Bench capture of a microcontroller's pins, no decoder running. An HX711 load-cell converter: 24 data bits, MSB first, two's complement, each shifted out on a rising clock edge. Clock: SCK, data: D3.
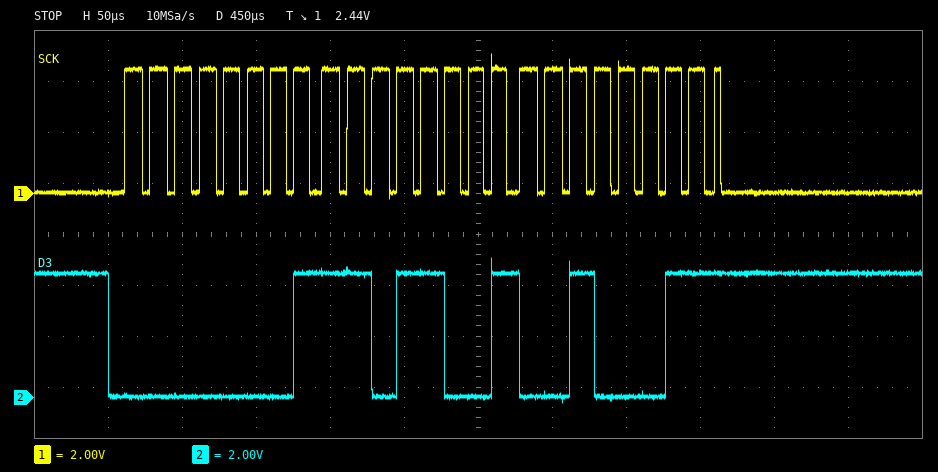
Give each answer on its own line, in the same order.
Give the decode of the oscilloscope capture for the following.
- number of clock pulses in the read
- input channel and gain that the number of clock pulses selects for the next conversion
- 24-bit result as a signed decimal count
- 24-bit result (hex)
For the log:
25
channel A, gain 128
121123
0x01D923
